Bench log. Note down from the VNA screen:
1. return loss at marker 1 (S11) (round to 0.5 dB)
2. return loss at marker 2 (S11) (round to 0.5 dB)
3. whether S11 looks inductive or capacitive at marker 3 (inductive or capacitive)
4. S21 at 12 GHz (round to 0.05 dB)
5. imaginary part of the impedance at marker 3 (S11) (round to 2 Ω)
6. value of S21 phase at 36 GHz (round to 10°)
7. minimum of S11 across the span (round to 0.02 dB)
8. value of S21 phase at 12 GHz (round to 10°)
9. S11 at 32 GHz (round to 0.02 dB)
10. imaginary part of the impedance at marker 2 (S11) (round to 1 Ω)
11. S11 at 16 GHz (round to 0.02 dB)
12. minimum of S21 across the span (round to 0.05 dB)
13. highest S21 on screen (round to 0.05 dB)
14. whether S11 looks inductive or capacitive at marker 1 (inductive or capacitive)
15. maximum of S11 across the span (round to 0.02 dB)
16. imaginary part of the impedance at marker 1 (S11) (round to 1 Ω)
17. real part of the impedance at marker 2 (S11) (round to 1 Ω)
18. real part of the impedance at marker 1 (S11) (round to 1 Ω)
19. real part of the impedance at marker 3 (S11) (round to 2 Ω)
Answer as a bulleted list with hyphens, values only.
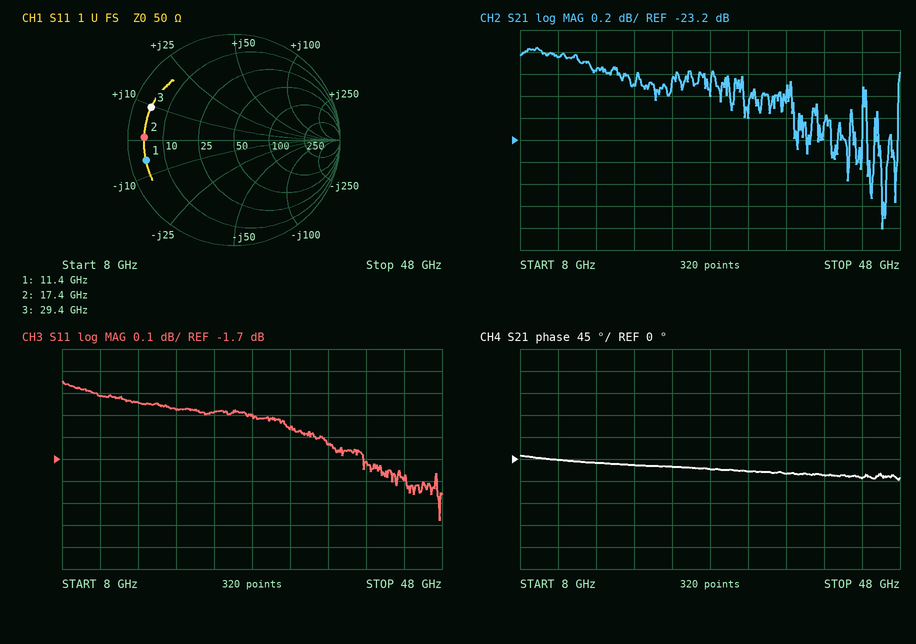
- 1.5 dB
- 1.5 dB
- inductive
- -22.45 dB
- +10 Ω
- -30°
- -1.98 dB
- 0°
- -1.56 dB
- +1 Ω
- -1.44 dB
- -24.00 dB
- -22.35 dB
- capacitive
- -1.34 dB
- -6 Ω
- 4 Ω
- 4 Ω
- 4 Ω
